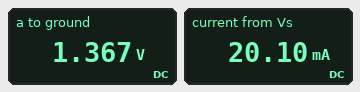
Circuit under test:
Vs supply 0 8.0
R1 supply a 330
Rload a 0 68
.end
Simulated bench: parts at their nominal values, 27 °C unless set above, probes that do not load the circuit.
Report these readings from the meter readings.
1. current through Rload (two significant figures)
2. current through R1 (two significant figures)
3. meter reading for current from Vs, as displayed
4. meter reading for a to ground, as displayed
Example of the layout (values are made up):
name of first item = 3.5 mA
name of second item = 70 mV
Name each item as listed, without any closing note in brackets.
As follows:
current through Rload = 20 mA
current through R1 = 20 mA
meter reading for current from Vs, as displayed = 20.10 mA
meter reading for a to ground, as displayed = 1.367 V
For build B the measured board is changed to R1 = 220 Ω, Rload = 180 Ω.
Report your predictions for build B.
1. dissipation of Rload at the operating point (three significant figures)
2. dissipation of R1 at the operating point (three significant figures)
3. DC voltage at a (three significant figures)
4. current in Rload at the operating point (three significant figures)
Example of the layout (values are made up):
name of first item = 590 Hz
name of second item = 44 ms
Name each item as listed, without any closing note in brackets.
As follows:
dissipation of Rload at the operating point = 72.0 mW
dissipation of R1 at the operating point = 88.0 mW
DC voltage at a = 3.60 V
current in Rload at the operating point = 20.0 mA
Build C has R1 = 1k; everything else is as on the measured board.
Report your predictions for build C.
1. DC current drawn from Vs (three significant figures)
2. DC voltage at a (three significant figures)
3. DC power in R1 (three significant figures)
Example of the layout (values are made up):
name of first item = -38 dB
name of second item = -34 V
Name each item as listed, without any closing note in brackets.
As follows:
DC current drawn from Vs = 7.49 mA
DC voltage at a = 509 mV
DC power in R1 = 56.1 mW
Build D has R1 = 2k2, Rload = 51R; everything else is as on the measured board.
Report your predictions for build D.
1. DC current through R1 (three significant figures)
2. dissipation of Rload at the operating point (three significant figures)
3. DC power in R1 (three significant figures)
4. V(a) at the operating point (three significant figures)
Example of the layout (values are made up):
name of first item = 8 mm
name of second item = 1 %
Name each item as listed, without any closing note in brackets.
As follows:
DC current through R1 = 3.55 mA
dissipation of Rload at the operating point = 644 µW
DC power in R1 = 27.8 mW
V(a) at the operating point = 181 mV
